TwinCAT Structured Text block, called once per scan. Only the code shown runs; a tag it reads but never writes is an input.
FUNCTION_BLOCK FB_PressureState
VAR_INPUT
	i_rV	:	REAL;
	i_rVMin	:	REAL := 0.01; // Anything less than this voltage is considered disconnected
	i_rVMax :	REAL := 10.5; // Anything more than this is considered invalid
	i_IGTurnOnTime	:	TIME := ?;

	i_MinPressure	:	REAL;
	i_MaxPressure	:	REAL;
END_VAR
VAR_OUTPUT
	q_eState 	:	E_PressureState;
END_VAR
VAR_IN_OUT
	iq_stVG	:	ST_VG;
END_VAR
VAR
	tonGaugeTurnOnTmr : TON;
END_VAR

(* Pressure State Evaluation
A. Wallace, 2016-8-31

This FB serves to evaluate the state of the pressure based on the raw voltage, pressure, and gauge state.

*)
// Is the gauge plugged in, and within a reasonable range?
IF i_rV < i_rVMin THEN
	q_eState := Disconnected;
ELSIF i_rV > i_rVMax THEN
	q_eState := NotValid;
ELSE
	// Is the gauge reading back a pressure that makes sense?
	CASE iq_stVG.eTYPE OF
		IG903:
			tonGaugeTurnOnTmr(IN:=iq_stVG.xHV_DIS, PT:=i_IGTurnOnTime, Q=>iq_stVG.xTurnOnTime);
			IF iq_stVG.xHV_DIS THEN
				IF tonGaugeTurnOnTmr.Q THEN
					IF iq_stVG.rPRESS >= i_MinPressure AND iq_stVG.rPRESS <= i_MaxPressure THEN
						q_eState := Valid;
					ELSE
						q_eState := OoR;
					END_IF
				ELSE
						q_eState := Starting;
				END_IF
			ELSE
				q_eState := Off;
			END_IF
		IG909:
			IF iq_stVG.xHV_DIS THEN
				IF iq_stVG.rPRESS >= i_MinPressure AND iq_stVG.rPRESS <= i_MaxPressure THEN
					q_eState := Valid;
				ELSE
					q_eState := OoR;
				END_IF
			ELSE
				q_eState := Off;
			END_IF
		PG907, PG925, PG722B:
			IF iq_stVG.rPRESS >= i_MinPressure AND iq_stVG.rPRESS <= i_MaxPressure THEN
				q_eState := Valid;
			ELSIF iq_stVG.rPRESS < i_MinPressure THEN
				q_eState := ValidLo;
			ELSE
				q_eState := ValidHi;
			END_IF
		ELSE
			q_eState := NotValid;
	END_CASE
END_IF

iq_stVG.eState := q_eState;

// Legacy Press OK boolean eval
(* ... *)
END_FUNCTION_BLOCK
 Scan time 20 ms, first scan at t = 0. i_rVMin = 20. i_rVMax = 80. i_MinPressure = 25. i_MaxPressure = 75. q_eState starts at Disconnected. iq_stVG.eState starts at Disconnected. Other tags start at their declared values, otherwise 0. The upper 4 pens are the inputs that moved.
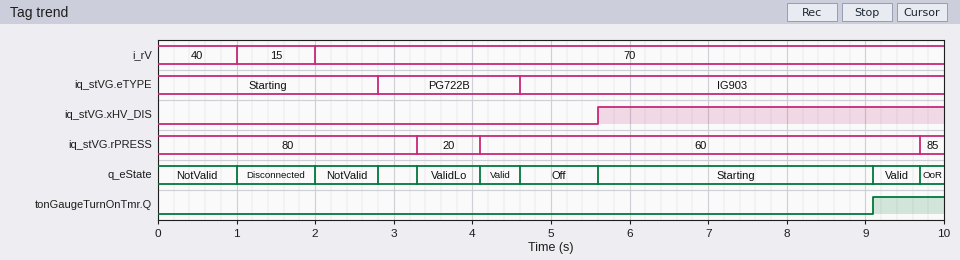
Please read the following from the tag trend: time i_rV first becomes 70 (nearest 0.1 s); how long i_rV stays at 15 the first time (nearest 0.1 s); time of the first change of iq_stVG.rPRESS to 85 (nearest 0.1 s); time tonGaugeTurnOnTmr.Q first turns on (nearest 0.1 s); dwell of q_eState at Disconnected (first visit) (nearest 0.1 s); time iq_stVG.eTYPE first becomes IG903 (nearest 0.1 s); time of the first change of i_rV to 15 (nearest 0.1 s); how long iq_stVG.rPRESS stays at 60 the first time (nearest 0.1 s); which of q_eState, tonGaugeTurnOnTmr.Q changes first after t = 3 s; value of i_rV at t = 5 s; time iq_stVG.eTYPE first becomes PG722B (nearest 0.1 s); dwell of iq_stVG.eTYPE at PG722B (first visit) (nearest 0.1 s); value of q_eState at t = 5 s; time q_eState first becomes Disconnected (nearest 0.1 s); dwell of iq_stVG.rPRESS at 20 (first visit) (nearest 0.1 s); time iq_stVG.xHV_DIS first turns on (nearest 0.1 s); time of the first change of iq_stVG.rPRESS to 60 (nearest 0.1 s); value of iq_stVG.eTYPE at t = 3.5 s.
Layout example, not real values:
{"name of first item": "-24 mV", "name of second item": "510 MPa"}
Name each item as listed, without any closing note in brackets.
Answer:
{"time i_rV first becomes 70": "2.0 s", "how long i_rV stays at 15 the first time": "1.0 s", "time of the first change of iq_stVG.rPRESS to 85": "9.7 s", "time tonGaugeTurnOnTmr.Q first turns on": "9.1 s", "dwell of q_eState at Disconnected (first visit)": "1.0 s", "time iq_stVG.eTYPE first becomes IG903": "4.6 s", "time of the first change of i_rV to 15": "1.0 s", "how long iq_stVG.rPRESS stays at 60 the first time": "5.6 s", "which of q_eState, tonGaugeTurnOnTmr.Q changes first after t = 3 s": "q_eState", "value of i_rV at t = 5 s": "70", "time iq_stVG.eTYPE first becomes PG722B": "2.8 s", "dwell of iq_stVG.eTYPE at PG722B (first visit)": "1.8 s", "value of q_eState at t = 5 s": "Off", "time q_eState first becomes Disconnected": "1.0 s", "dwell of iq_stVG.rPRESS at 20 (first visit)": "0.8 s", "time iq_stVG.xHV_DIS first turns on": "5.6 s", "time of the first change of iq_stVG.rPRESS to 60": "4.1 s", "value of iq_stVG.eTYPE at t = 3.5 s": "PG722B"}
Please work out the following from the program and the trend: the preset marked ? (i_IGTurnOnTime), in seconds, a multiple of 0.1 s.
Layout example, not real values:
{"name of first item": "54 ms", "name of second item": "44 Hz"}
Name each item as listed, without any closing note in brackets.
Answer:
{"the preset marked ? (i_IGTurnOnTime), in seconds, a multiple of 0.1 s": "3.5 s"}
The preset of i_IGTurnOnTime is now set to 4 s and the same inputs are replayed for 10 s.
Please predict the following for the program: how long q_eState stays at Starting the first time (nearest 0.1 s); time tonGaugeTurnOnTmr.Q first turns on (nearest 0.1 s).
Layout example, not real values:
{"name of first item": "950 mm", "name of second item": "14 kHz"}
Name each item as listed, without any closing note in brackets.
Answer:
{"how long q_eState stays at Starting the first time": "4.0 s", "time tonGaugeTurnOnTmr.Q first turns on": "9.6 s"}
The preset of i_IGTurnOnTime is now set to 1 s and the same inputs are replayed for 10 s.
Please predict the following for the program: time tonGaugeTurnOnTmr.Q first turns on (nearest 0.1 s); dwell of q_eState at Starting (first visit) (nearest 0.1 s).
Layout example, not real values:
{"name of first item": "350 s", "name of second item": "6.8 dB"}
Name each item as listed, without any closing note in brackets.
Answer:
{"time tonGaugeTurnOnTmr.Q first turns on": "6.6 s", "dwell of q_eState at Starting (first visit)": "1.0 s"}
